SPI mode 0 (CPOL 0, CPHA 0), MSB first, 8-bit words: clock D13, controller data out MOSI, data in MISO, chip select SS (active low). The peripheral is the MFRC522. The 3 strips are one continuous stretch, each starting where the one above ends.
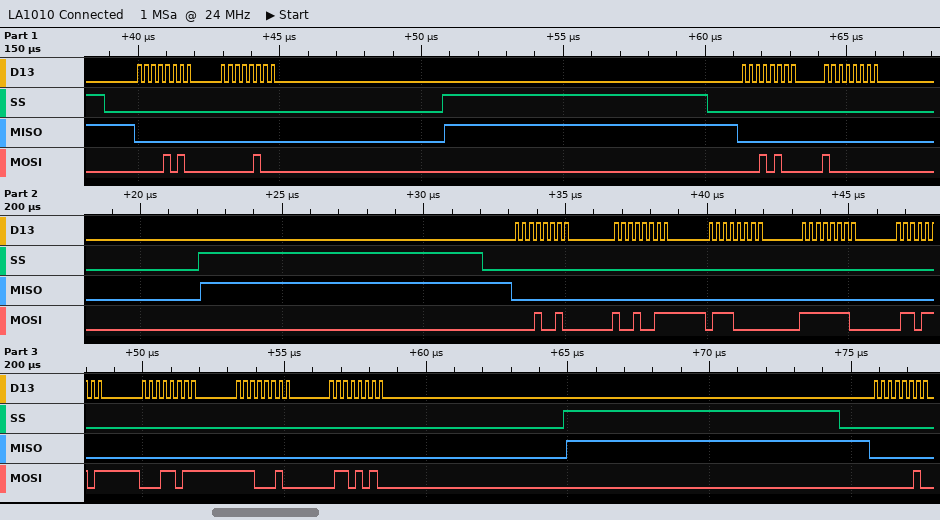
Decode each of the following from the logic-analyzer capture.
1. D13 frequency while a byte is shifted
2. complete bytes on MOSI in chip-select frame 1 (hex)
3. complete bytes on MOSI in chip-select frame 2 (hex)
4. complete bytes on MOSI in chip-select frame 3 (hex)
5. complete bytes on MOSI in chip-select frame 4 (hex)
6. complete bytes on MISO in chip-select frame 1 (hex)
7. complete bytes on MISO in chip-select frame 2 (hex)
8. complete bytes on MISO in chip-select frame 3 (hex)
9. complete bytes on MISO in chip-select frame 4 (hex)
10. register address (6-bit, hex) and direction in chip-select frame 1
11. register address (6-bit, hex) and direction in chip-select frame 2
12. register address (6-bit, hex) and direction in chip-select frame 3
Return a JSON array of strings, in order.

["4 MHz", "0A 04", "14 80", "12 93 70 FE 6D 1B E2 6A", "02", "00 00", "00 00", "00 00 00 00 00 00 00 00", "00", "0x05 write", "0x0A write", "0x09 write"]
